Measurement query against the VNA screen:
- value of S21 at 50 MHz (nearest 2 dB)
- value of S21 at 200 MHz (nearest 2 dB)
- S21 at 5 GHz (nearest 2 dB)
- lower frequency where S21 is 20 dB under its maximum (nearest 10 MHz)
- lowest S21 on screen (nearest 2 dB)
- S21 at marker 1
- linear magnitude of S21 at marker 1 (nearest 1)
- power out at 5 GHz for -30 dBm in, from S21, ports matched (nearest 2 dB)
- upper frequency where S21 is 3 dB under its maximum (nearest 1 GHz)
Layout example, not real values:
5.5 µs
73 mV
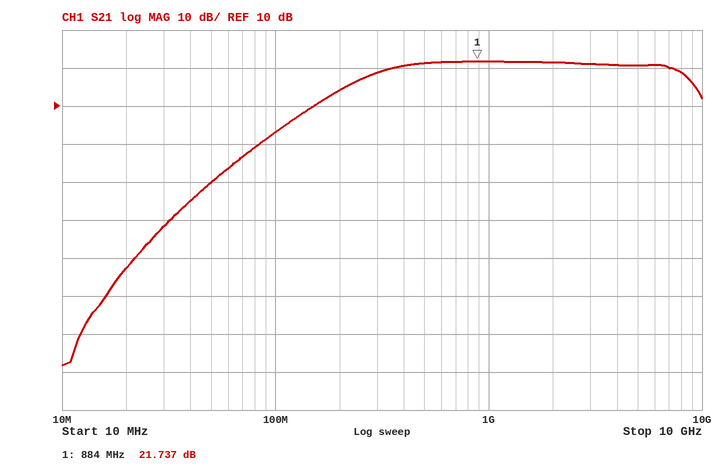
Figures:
-10 dB
14 dB
20 dB
90 MHz
-58 dB
21.737 dB
12
-10 dBm
8 GHz
